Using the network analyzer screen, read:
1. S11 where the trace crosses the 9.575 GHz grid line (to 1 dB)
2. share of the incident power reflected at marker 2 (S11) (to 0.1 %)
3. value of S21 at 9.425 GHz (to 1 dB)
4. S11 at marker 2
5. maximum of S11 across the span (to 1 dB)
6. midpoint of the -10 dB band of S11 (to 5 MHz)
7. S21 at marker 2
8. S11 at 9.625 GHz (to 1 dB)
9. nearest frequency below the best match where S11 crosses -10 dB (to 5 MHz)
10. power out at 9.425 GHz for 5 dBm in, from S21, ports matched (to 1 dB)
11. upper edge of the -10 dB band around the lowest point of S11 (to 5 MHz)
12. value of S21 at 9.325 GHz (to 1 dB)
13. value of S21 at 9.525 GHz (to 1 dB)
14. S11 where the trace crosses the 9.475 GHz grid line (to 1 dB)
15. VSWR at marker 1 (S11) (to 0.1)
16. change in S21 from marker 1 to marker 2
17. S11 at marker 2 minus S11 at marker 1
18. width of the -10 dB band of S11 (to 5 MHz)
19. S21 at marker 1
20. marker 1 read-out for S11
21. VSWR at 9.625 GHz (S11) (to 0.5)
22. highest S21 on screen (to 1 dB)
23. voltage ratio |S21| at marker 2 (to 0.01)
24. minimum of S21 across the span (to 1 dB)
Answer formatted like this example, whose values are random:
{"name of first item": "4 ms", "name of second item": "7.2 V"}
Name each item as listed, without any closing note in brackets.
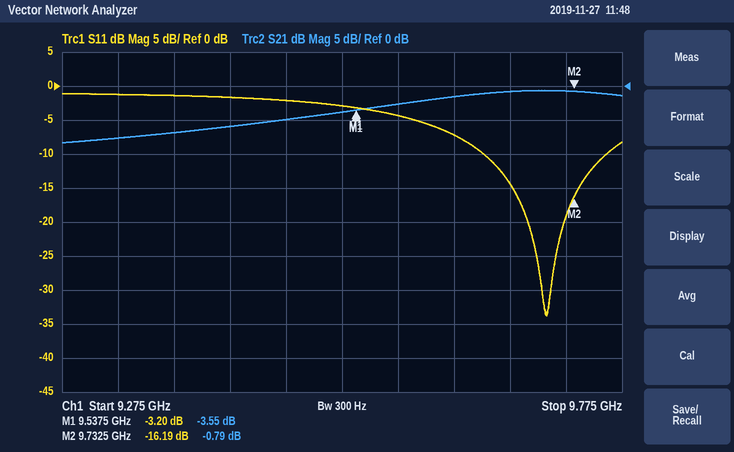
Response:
{"S11 where the trace crosses the 9.575 GHz grid line": "-4 dB", "share of the incident power reflected at marker 2 (S11)": "2.4 %", "value of S21 at 9.425 GHz": "-6 dB", "S11 at marker 2": "-16.19 dB", "maximum of S11 across the span": "-1 dB", "midpoint of the -10 dB band of S11": "9.705 GHz", "S21 at marker 2": "-0.79 dB", "S11 at 9.625 GHz": "-7 dB", "nearest frequency below the best match where S11 crosses -10 dB": "9.650 GHz", "power out at 9.425 GHz for 5 dBm in, from S21, ports matched": "-1 dBm", "upper edge of the -10 dB band around the lowest point of S11": "9.760 GHz", "value of S21 at 9.325 GHz": "-8 dB", "value of S21 at 9.525 GHz": "-4 dB", "S11 where the trace crosses the 9.475 GHz grid line": "-2 dB", "VSWR at marker 1 (S11)": "5.5", "change in S21 from marker 1 to marker 2": "2.76 dB", "S11 at marker 2 minus S11 at marker 1": "-12.99 dB", "width of the -10 dB band of S11": "110 MHz", "S21 at marker 1": "-3.55 dB", "marker 1 read-out for S11": "-3.20 dB", "VSWR at 9.625 GHz (S11)": "2.5", "highest S21 on screen": "-1 dB", "voltage ratio |S21| at marker 2": "0.91", "minimum of S21 across the span": "-8 dB"}
